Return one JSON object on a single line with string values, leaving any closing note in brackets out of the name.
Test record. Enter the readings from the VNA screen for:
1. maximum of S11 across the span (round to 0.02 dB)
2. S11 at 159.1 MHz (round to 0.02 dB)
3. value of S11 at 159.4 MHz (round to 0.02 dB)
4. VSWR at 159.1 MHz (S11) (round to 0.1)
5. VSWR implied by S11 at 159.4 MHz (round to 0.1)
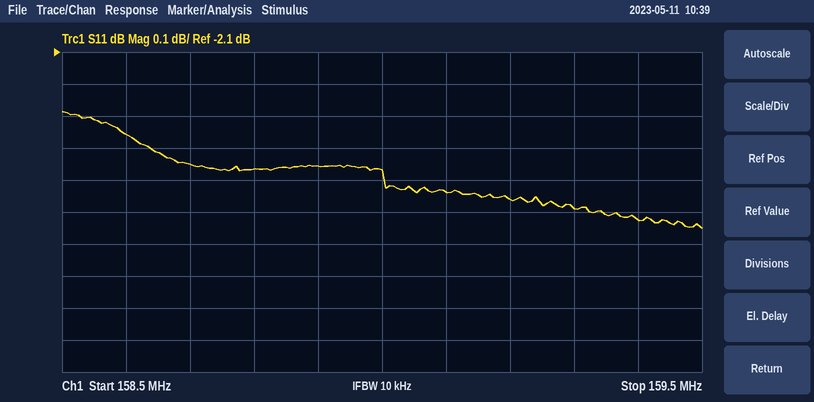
{"maximum of S11 across the span": "-2.28 dB", "S11 at 159.1 MHz": "-2.54 dB", "value of S11 at 159.4 MHz": "-2.62 dB", "VSWR at 159.1 MHz (S11)": "6.9", "VSWR implied by S11 at 159.4 MHz": "6.7"}
